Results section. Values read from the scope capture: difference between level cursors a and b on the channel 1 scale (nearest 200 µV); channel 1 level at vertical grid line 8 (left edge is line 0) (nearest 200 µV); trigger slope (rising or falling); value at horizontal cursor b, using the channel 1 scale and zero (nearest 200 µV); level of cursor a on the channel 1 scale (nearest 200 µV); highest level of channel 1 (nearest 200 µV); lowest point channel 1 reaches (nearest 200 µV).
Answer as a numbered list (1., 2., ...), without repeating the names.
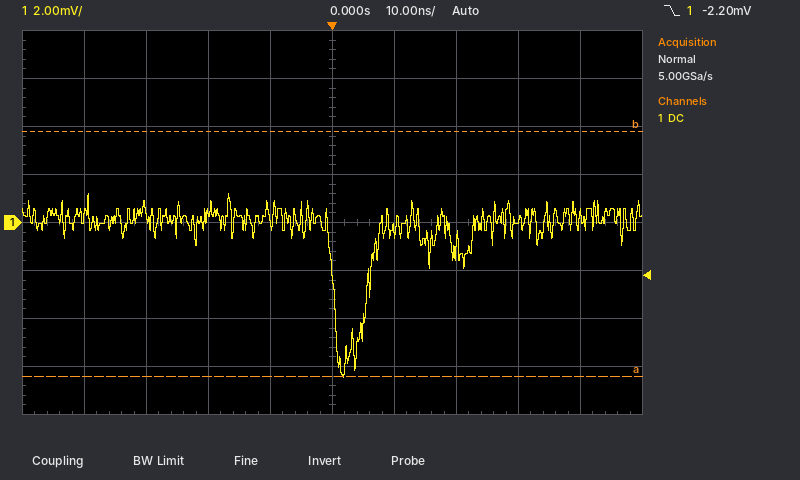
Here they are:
1. 10.2 mV
2. 200 µV
3. falling
4. 3.8 mV
5. -6.4 mV
6. 1.2 mV
7. -6.4 mV
